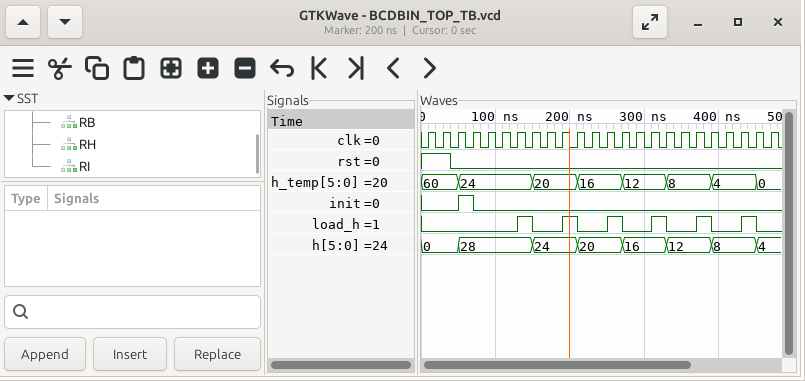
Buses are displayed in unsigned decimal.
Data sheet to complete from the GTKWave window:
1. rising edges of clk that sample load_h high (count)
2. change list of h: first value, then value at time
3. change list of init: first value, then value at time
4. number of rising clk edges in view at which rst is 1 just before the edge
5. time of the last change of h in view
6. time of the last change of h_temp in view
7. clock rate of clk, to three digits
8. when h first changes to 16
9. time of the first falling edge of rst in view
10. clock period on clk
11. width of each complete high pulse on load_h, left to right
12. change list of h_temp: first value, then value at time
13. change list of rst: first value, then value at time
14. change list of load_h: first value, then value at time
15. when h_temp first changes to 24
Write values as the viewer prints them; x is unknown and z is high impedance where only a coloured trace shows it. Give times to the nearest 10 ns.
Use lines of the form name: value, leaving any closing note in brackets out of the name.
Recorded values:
rising edges of clk that sample load_h high: 6
change list of h: first value, then value at time: 0, 28 at 50 ns, 24 at 150 ns, 20 at 210 ns, 16 at 270 ns, 12 at 330 ns, 8 at 390 ns, 4 at 450 ns
change list of init: first value, then value at time: 0, 1 at 50 ns, 0 at 70 ns
number of rising clk edges in view at which rst is 1 just before the edge: 2
time of the last change of h in view: 450 ns
time of the last change of h_temp in view: 450 ns
clock rate of clk, to three digits: 50.0 MHz
when h first changes to 16: 270 ns
time of the first falling edge of rst in view: 40 ns
clock period on clk: 20 ns
width of each complete high pulse on load_h, left to right: 20 ns, 20 ns, 20 ns, 20 ns, 20 ns, 20 ns
change list of h_temp: first value, then value at time: 60, 24 at 50 ns, 20 at 150 ns, 16 at 210 ns, 12 at 270 ns, 8 at 330 ns, 4 at 390 ns, 0 at 450 ns
change list of rst: first value, then value at time: 1, 0 at 40 ns
change list of load_h: first value, then value at time: 0, 1 at 130 ns, 0 at 150 ns, 1 at 190 ns, 0 at 210 ns, 1 at 250 ns, 0 at 270 ns, 1 at 310 ns, 0 at 330 ns, 1 at 370 ns, 0 at 390 ns, 1 at 430 ns, 0 at 450 ns
when h_temp first changes to 24: 50 ns
